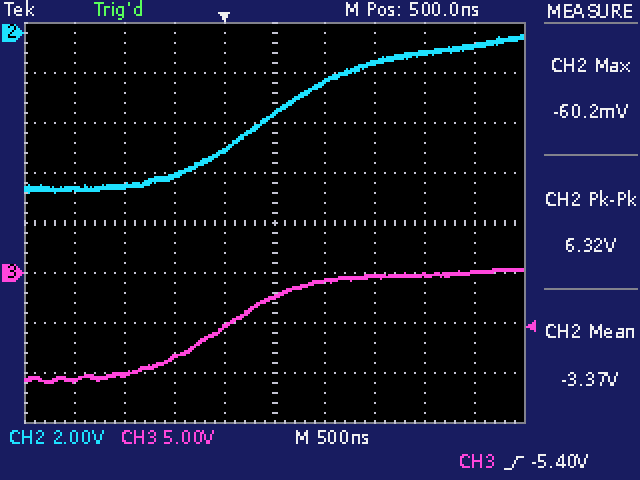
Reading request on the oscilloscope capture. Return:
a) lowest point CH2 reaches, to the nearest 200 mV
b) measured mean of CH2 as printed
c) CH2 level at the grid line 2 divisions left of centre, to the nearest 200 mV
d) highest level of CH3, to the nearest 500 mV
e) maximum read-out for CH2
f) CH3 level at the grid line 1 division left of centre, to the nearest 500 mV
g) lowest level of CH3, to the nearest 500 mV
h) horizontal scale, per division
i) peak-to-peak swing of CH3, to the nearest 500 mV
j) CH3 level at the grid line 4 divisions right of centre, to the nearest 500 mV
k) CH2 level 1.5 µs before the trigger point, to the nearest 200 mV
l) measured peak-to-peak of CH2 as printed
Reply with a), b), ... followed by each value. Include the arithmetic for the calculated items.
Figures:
a) -6.4 V
b) -3.37 V
c) -5.8 V
d) 500 mV
e) -60.2 mV
f) -5.5 V
g) -11.0 V
h) 500 ns
i) 500 mV − (-11.0 V) = 11.5 V
j) 0.0 V
k) -6.2 V
l) 6.32 V
